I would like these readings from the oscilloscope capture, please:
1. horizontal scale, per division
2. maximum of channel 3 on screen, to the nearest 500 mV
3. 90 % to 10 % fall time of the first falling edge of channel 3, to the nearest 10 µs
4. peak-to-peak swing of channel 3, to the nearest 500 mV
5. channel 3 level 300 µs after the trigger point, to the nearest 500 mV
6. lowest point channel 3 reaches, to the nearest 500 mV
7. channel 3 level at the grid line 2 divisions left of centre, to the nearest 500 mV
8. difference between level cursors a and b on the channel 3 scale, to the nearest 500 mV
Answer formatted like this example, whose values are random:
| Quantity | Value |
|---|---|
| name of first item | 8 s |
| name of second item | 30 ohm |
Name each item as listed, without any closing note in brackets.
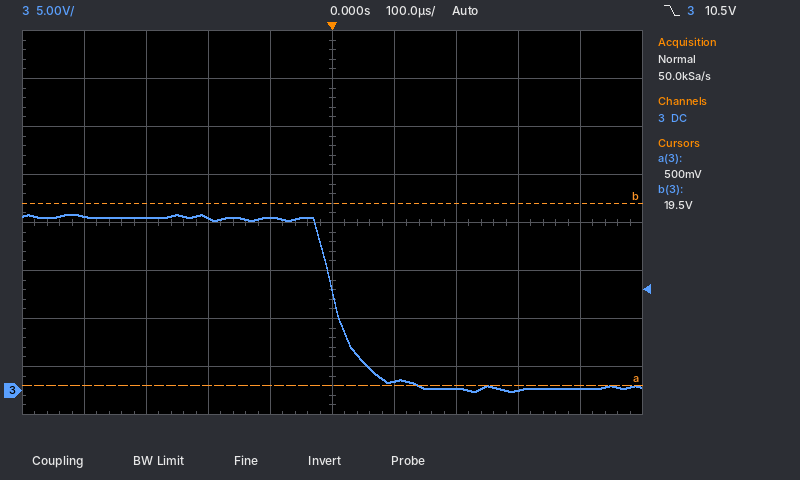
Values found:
| Quantity | Value |
|---|---|
| horizontal scale, per division | 100 µs |
| maximum of channel 3 on screen, to the nearest 500 mV | 18.5 V |
| 90 % to 10 % fall time of the first falling edge of channel 3, to the nearest 10 µs | 90 µs |
| peak-to-peak swing of channel 3, to the nearest 500 mV | 18.5 V |
| channel 3 level 300 µs after the trigger point, to the nearest 500 mV | 0.0 V |
| lowest point channel 3 reaches, to the nearest 500 mV | 0.0 V |
| channel 3 level at the grid line 2 divisions left of centre, to the nearest 500 mV | 18.0 V |
| difference between level cursors a and b on the channel 3 scale, to the nearest 500 mV | 19.0 V |
